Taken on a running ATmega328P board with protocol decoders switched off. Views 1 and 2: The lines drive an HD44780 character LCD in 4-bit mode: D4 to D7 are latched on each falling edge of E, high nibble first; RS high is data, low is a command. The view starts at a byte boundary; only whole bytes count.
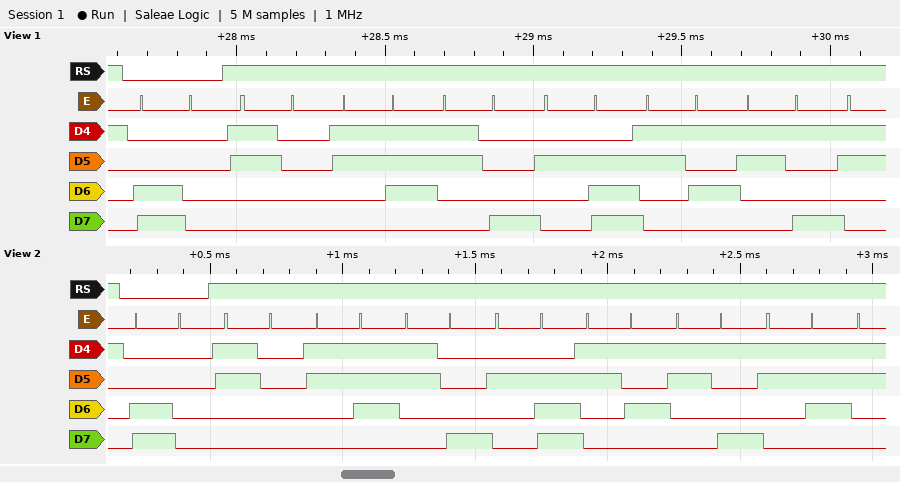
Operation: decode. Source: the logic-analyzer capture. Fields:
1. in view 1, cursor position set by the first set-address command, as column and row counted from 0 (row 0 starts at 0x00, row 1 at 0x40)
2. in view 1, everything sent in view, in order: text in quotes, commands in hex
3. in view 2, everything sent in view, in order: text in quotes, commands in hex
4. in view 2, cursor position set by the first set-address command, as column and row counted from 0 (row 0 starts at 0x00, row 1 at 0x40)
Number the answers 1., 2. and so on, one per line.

1. column 0, row 1
2. 0xC0 "078.59"
3. 0xC0 "078.597"
4. column 0, row 1
